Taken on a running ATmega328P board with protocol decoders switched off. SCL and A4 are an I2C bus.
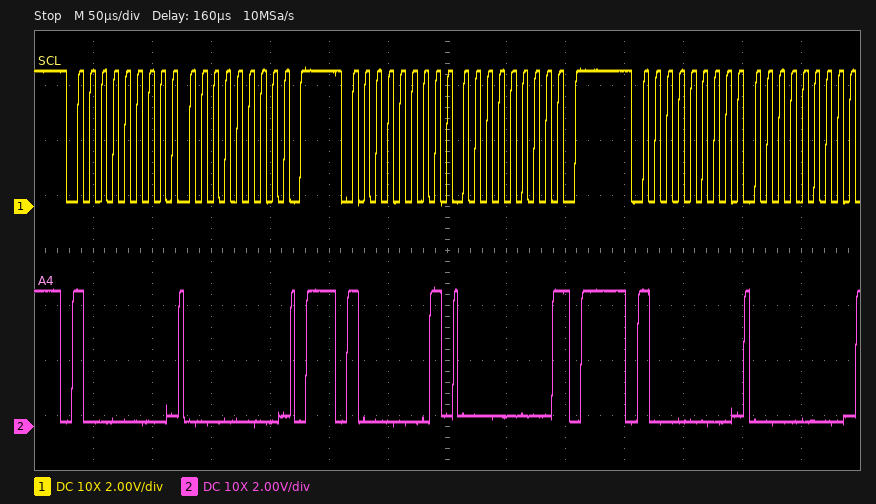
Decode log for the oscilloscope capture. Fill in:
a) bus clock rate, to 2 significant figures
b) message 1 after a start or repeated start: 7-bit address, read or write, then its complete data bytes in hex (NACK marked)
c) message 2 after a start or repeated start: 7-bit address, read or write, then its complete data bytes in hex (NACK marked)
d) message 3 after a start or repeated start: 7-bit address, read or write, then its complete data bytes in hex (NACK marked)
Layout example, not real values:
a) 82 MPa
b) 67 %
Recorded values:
a) 100 kHz
b) 0x40 write: 00
c) 0x40 read: 00 NACK
d) 0x40 write: 00
